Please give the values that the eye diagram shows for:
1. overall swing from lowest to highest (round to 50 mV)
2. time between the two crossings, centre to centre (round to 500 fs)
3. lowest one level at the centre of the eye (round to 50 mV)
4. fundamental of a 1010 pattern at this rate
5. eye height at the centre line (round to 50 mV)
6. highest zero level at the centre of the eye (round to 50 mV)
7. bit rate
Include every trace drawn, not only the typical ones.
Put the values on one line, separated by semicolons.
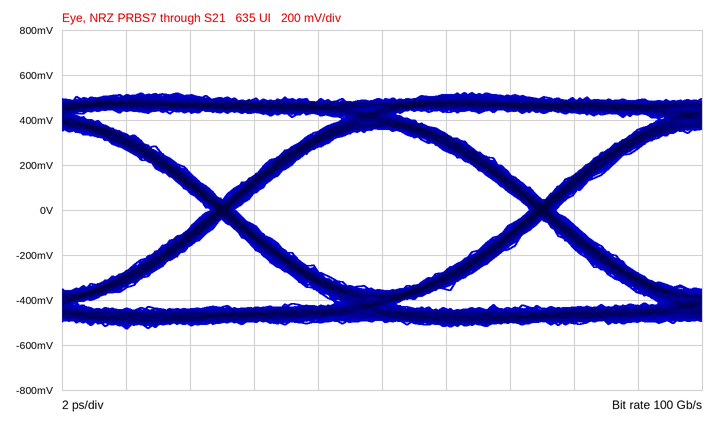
1.05 V; 10.0 ps; 350 mV; 50 GHz; 700 mV; -350 mV; 100 Gb/s
